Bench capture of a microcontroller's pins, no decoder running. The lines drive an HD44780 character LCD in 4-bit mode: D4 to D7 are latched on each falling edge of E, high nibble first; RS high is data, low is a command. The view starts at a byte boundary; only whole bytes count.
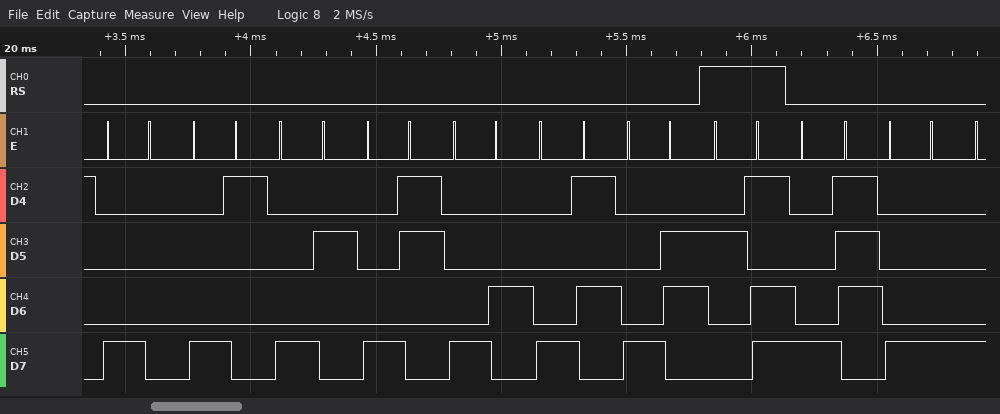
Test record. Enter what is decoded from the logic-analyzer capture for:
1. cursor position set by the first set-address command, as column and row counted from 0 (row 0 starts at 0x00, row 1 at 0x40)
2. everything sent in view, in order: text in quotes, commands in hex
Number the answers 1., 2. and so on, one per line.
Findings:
1. column 0, row 0
2. 0x80 0x81 0x82 0x83 0x84 0x85 0x86 "-" 0x87 0x88
